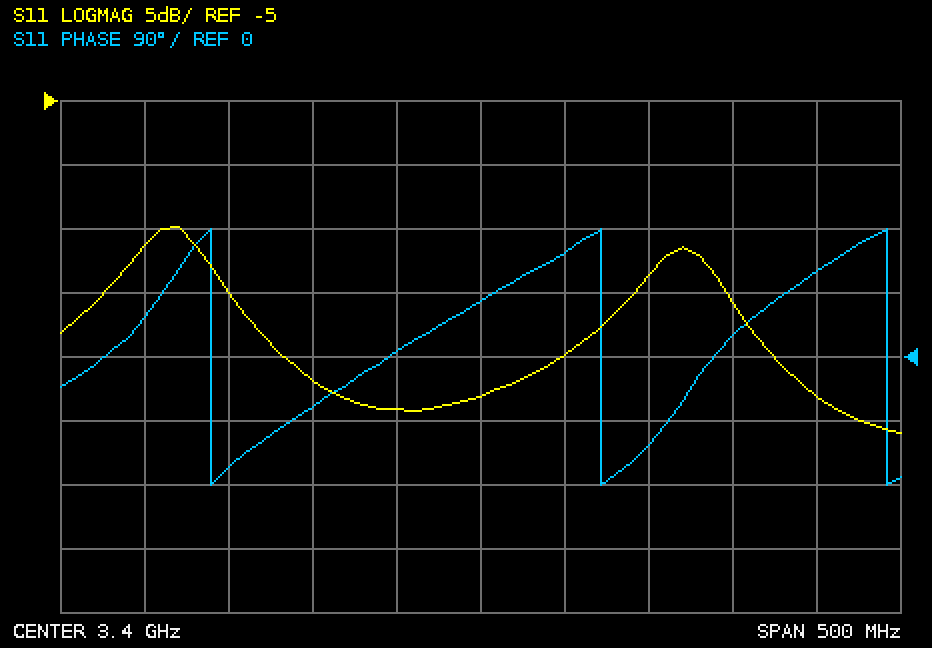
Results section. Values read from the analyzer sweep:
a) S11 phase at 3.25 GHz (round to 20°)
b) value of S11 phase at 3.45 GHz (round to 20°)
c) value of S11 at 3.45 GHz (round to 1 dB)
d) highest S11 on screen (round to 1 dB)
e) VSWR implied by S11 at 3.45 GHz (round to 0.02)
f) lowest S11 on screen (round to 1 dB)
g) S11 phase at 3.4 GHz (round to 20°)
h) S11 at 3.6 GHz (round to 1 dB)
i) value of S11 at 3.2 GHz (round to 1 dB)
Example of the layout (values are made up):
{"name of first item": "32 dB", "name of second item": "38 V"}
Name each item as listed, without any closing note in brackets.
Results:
{"S11 phase at 3.25 GHz": "-160°", "value of S11 phase at 3.45 GHz": "140°", "value of S11 at 3.45 GHz": "-25 dB", "highest S11 on screen": "-15 dB", "VSWR implied by S11 at 3.45 GHz": "1.12", "lowest S11 on screen": "-31 dB", "S11 phase at 3.4 GHz": "80°", "S11 at 3.6 GHz": "-28 dB", "value of S11 at 3.2 GHz": "-16 dB"}
